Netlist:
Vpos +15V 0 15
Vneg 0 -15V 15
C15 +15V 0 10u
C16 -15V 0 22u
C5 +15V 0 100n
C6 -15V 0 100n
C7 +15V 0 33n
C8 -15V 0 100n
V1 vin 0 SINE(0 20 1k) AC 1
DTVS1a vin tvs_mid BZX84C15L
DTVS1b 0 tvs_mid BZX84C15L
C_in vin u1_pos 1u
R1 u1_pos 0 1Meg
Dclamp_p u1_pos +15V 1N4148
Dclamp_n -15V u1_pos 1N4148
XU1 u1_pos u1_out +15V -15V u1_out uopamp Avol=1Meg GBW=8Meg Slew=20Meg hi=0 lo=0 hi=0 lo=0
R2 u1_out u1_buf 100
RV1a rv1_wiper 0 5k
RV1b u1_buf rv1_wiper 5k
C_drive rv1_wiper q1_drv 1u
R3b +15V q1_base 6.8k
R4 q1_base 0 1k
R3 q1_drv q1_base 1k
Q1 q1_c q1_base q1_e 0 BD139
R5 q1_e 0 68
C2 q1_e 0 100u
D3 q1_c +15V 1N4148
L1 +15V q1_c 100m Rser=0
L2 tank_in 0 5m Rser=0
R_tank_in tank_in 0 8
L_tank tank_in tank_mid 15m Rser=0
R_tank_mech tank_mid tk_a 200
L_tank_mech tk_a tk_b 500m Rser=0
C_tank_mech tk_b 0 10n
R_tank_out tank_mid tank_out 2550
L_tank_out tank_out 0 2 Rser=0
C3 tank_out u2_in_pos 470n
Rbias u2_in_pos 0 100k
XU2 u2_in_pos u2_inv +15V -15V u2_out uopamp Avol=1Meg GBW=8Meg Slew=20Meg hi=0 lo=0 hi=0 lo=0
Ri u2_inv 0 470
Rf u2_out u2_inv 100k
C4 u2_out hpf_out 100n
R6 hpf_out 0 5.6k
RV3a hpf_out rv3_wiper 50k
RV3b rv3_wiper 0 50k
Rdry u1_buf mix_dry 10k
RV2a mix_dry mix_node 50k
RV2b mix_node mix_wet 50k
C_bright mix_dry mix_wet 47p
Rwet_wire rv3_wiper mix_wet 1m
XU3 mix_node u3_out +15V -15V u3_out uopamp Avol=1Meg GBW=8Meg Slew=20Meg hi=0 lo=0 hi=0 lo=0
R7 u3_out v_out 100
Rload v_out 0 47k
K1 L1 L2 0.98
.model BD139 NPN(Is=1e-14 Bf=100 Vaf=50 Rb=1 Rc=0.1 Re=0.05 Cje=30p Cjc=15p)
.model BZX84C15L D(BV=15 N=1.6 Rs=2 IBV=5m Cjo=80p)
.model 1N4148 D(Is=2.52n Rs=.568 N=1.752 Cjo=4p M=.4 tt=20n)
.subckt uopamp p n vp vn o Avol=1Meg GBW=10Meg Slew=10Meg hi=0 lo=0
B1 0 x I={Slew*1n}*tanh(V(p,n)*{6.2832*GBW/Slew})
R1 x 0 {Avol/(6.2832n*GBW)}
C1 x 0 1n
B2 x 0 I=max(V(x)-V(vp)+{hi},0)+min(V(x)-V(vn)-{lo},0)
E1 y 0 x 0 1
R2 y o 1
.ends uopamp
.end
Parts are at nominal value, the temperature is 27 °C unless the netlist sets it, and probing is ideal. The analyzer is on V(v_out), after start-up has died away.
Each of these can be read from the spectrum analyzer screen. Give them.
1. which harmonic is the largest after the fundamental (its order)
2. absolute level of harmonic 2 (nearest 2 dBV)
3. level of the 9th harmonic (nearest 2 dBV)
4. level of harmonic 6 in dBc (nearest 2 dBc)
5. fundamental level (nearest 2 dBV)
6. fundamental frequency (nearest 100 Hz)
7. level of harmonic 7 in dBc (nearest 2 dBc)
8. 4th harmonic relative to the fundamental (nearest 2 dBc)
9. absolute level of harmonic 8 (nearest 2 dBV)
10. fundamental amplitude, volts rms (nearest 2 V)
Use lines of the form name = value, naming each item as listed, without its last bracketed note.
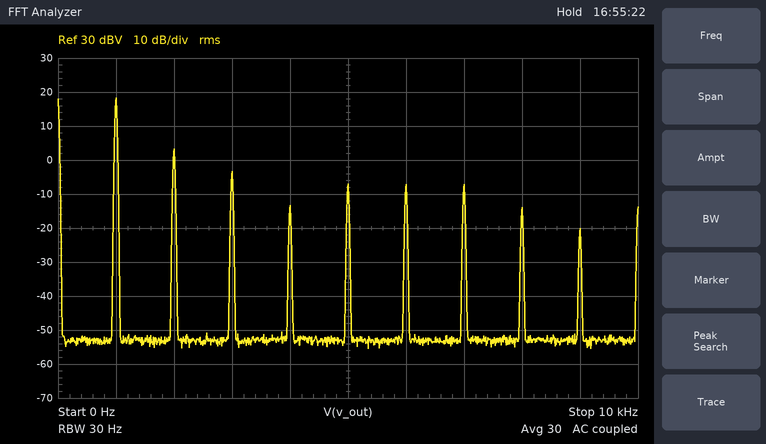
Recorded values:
which harmonic is the largest after the fundamental = 2
absolute level of harmonic 2 = 4 dBV
level of the 9th harmonic = -20 dBV
level of harmonic 6 in dBc = -26 dBc
fundamental level = 18 dBV
fundamental frequency = 1.0 kHz
level of harmonic 7 in dBc = -26 dBc
4th harmonic relative to the fundamental = -32 dBc
absolute level of harmonic 8 = -14 dBV
fundamental amplitude, volts rms = 8 V
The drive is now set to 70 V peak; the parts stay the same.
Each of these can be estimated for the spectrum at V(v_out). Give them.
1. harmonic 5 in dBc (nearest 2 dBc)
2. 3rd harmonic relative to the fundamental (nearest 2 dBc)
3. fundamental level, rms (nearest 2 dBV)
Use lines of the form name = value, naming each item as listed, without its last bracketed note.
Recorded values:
harmonic 5 in dBc = -18 dBc
3rd harmonic relative to the fundamental = -12 dBc
fundamental level, rms = 18 dBV
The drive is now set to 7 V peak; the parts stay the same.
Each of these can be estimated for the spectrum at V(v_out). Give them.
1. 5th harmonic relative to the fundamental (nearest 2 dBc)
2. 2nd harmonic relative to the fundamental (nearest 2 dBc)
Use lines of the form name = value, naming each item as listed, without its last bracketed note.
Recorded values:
5th harmonic relative to the fundamental = -24 dBc
2nd harmonic relative to the fundamental = -10 dBc
